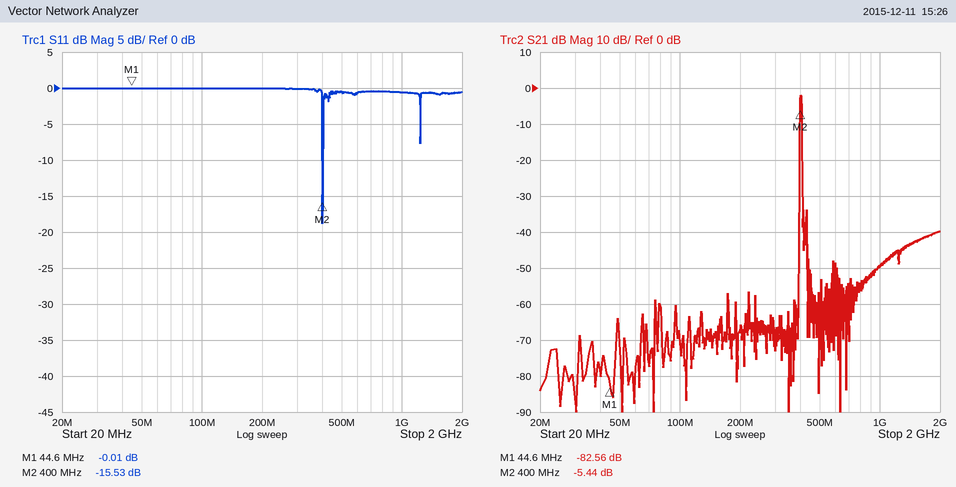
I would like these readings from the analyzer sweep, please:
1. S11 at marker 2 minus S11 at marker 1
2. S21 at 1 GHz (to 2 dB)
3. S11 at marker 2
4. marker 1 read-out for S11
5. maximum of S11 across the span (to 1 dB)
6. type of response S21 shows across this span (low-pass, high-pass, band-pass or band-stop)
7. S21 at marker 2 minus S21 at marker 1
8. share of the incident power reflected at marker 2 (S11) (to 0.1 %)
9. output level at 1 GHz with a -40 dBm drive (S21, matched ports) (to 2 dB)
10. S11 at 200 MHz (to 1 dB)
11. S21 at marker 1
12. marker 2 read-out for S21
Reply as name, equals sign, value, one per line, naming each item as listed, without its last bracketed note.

S11 at marker 2 minus S11 at marker 1 = -15.52 dB
S21 at 1 GHz = -50 dB
S11 at marker 2 = -15.53 dB
marker 1 read-out for S11 = -0.01 dB
maximum of S11 across the span = 0 dB
type of response S21 shows across this span = band-pass
S21 at marker 2 minus S21 at marker 1 = 77.12 dB
share of the incident power reflected at marker 2 (S11) = 2.8 %
output level at 1 GHz with a -40 dBm drive (S21, matched ports) = -90 dBm
S11 at 200 MHz = 0 dB
S21 at marker 1 = -82.56 dB
marker 2 read-out for S21 = -5.44 dB
